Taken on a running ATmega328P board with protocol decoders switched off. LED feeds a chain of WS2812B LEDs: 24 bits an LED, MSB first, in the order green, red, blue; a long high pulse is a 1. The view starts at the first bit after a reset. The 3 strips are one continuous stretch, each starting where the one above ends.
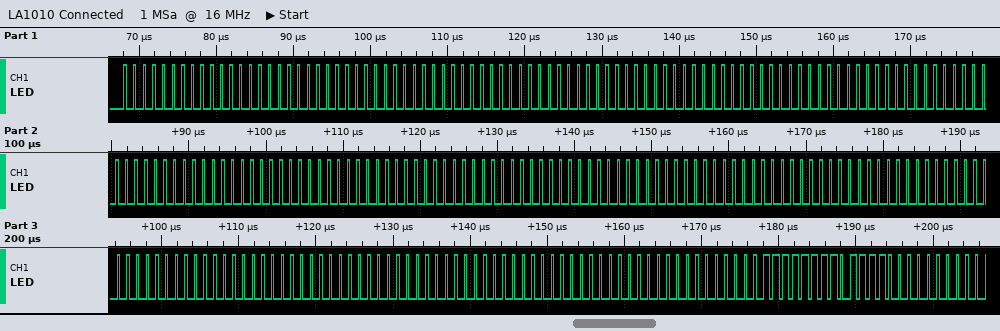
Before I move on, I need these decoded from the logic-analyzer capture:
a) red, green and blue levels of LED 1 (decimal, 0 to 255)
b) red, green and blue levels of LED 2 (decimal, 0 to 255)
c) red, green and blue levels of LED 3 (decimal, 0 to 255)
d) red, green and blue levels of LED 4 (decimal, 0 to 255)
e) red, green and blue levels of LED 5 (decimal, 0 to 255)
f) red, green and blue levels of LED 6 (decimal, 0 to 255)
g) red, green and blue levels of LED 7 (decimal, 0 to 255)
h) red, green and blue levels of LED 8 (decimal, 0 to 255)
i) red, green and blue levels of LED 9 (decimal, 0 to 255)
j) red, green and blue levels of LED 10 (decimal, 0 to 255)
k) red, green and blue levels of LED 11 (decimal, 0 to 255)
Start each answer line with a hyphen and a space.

- 0, 0, 0
- 0, 0, 0
- 0, 0, 0
- 0, 0, 0
- 0, 0, 0
- 0, 0, 0
- 0, 0, 0
- 0, 0, 0
- 0, 0, 0
- 0, 0, 0
- 255, 0, 120
